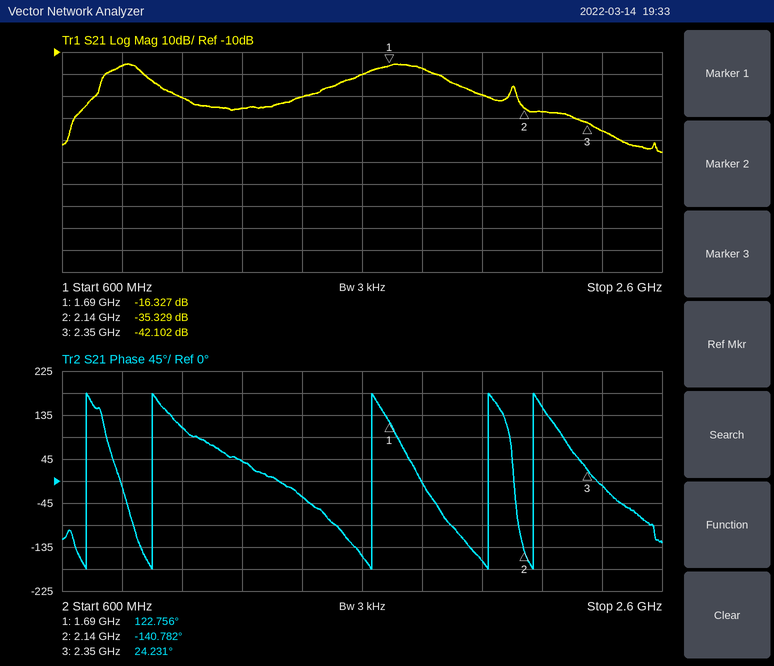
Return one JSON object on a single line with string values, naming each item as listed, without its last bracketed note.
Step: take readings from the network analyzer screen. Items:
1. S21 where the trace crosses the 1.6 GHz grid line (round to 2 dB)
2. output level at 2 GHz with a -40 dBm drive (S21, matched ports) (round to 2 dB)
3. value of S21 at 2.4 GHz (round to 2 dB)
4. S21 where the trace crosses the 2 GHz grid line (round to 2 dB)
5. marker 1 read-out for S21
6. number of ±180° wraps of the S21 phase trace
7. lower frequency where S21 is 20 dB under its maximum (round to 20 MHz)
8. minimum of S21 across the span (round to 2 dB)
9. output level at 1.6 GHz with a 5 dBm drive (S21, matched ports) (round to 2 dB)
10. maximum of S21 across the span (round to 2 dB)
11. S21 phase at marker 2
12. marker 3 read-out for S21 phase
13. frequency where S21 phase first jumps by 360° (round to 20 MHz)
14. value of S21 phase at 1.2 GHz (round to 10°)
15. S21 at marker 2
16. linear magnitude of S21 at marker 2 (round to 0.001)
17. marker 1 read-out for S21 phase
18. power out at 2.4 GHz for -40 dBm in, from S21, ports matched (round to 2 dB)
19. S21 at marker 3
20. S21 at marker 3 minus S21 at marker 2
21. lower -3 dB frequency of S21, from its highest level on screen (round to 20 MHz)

{"S21 where the trace crosses the 1.6 GHz grid line": "-20 dB", "output level at 2 GHz with a -40 dBm drive (S21, matched ports)": "-70 dBm", "value of S21 at 2.4 GHz": "-46 dB", "S21 where the trace crosses the 2 GHz grid line": "-30 dB", "marker 1 read-out for S21": "-16.327 dB", "number of ±180° wraps of the S21 phase trace": "5", "lower frequency where S21 is 20 dB under its maximum": "680 MHz", "minimum of S21 across the span": "-56 dB", "output level at 1.6 GHz with a 5 dBm drive (S21, matched ports)": "-16 dBm", "maximum of S21 across the span": "-16 dB", "S21 phase at marker 2": "-140.782°", "marker 3 read-out for S21 phase": "24.231°", "frequency where S21 phase first jumps by 360°": "680 MHz", "value of S21 phase at 1.2 GHz": "40°", "S21 at marker 2": "-35.329 dB", "linear magnitude of S21 at marker 2": "0.017", "marker 1 read-out for S21 phase": "122.756°", "power out at 2.4 GHz for -40 dBm in, from S21, ports matched": "-86 dBm", "S21 at marker 3": "-42.102 dB", "S21 at marker 3 minus S21 at marker 2": "-6.773 dB", "lower -3 dB frequency of S21, from its highest level on screen": "760 MHz"}
